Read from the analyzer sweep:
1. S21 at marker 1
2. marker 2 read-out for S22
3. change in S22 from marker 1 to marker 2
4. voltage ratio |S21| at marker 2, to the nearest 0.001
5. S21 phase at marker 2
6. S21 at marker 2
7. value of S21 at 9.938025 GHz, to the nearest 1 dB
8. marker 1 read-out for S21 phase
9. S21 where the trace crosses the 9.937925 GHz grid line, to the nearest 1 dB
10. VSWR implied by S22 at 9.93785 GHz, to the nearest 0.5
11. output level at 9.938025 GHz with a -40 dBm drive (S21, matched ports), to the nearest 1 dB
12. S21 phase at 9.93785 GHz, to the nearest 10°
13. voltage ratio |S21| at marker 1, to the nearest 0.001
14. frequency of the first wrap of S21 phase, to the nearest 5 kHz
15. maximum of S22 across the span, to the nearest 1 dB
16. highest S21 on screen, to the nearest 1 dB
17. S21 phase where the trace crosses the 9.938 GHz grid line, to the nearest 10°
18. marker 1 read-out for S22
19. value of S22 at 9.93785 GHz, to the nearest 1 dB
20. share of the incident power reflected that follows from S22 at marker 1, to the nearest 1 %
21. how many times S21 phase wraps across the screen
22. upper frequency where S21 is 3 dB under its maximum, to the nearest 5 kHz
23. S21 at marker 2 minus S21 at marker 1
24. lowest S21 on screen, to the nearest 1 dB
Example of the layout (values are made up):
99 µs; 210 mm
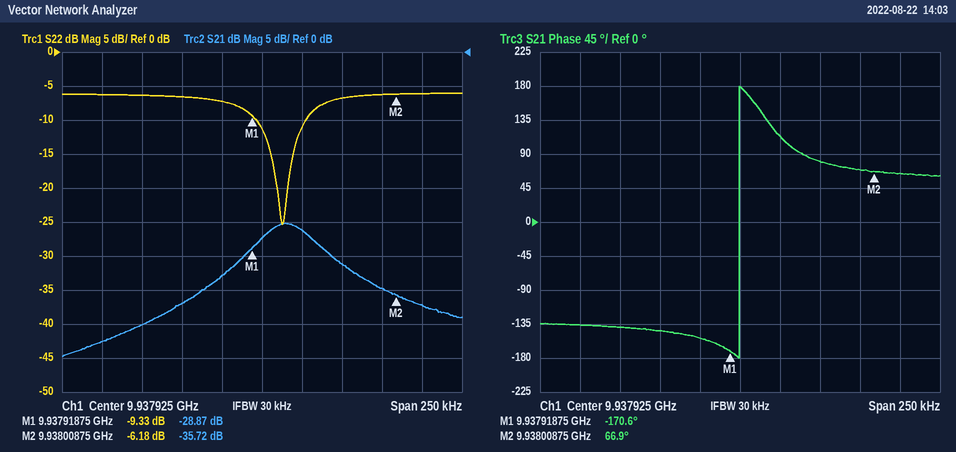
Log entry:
-28.87 dB; -6.18 dB; 3.15 dB; 0.016; 66.9°; -35.72 dB; -37 dB; -170.6°; -27 dB; 3.0; -77 dBm; -140°; 0.036; 9.937925 GHz; -6 dB; -25 dB; 70°; -9.33 dB; -6 dB; 12 %; 1; 9.937960 GHz; -6.85 dB; -45 dB
